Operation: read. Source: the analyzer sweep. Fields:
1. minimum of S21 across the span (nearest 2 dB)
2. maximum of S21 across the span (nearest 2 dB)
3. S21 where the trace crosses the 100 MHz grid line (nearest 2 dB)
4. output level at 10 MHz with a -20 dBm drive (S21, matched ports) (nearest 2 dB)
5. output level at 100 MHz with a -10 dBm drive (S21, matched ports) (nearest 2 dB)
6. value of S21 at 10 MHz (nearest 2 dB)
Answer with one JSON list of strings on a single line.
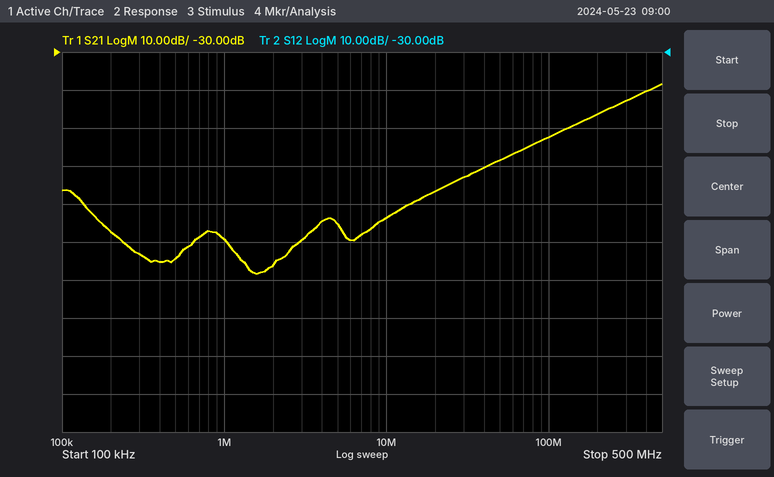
["-88 dB", "-38 dB", "-52 dB", "-94 dBm", "-62 dBm", "-74 dB"]
